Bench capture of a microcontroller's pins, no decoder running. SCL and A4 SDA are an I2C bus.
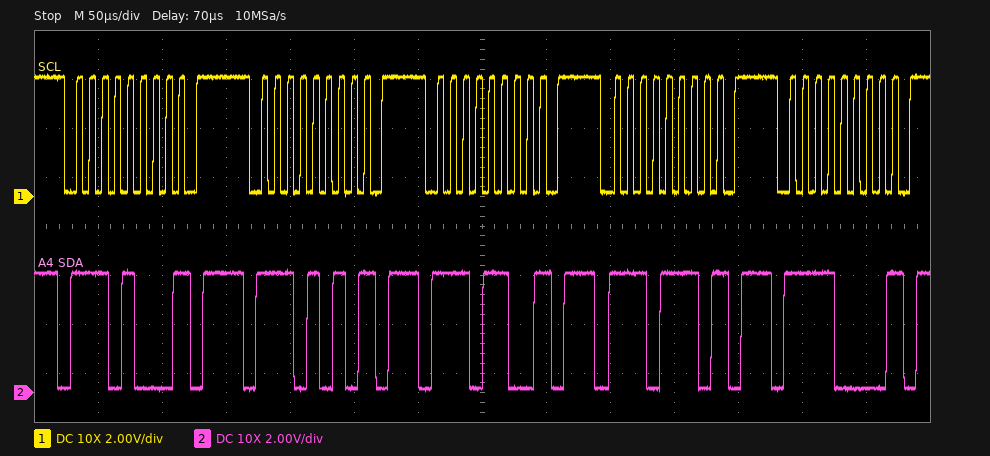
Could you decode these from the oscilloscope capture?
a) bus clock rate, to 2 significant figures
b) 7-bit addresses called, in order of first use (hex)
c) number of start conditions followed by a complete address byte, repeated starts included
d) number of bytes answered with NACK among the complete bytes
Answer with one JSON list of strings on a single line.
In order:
["100 kHz", "0x74 0x75 0x76 0x77 0x78", "5", "5"]
